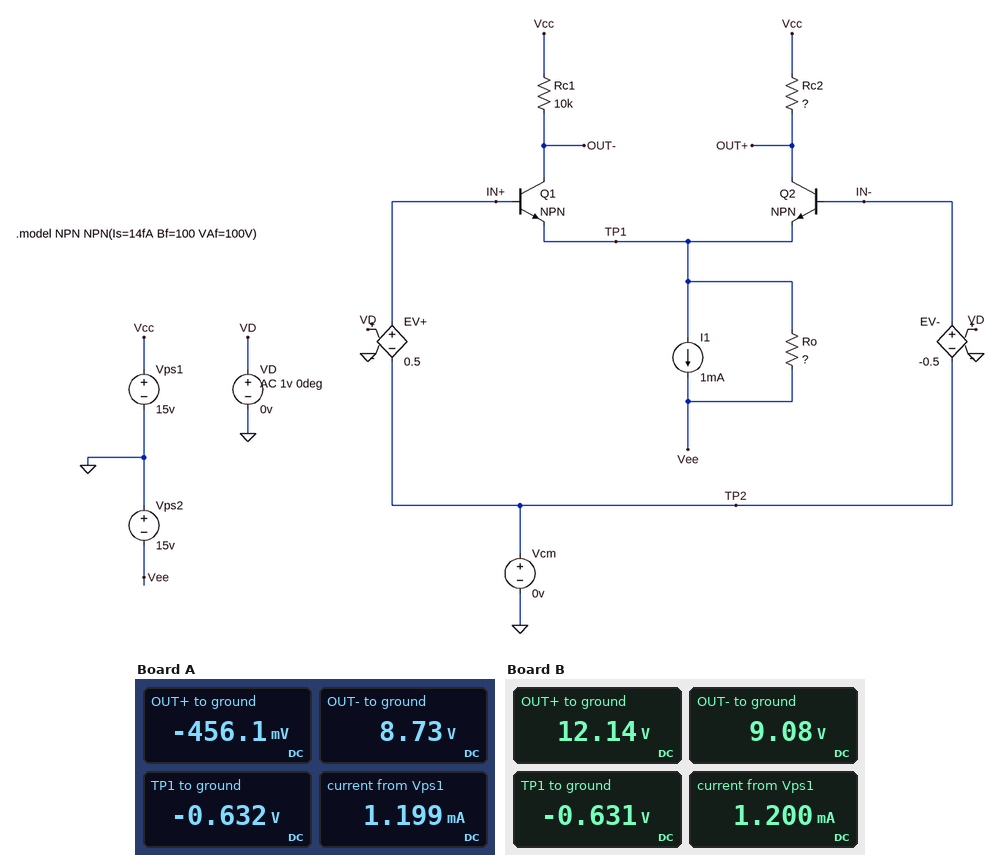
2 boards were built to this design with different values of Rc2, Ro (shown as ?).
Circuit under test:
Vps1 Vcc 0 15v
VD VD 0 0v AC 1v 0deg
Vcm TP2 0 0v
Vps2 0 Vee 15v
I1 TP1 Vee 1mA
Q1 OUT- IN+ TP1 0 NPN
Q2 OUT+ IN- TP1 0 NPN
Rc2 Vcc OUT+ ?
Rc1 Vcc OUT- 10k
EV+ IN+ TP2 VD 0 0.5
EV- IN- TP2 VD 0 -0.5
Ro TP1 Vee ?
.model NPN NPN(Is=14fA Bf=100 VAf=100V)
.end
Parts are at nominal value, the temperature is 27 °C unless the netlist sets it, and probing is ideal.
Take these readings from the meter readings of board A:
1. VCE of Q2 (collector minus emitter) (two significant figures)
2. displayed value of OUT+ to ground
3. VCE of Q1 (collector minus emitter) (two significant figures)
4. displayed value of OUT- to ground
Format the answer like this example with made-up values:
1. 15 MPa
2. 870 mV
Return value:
1. 180 mV
2. -456.1 mV
3. 9.4 V
4. 8.73 V
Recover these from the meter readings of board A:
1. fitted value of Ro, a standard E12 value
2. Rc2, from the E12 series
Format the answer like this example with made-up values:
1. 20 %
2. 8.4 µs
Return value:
1. 68 kΩ
2. 27 kΩ
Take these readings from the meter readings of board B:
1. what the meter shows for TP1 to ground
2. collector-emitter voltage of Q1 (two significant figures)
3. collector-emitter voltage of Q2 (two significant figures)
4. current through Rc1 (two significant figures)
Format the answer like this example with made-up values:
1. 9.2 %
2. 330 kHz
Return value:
1. -0.631 V
2. 9.7 V
3. 13 V
4. 590 µA
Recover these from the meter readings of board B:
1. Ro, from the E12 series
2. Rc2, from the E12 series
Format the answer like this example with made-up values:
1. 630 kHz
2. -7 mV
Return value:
1. 68 kΩ
2. 4.7 kΩ
